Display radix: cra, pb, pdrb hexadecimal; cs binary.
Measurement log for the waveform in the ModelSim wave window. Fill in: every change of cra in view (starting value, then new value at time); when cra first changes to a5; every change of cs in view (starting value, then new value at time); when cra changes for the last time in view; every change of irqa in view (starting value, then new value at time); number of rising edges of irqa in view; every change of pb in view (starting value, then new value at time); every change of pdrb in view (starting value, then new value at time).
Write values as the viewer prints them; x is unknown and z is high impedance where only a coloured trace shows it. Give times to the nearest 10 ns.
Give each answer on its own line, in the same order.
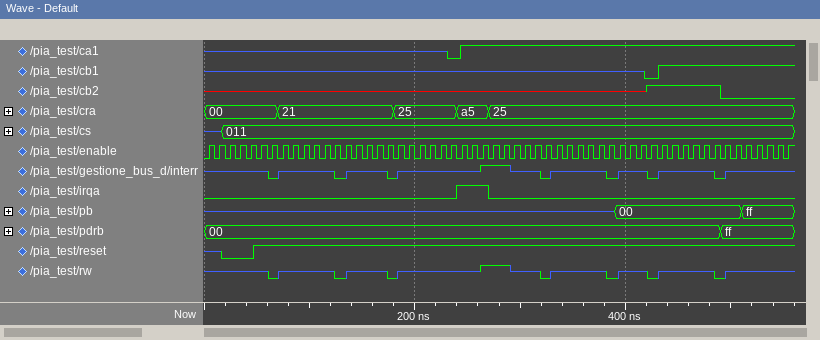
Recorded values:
00, 21 at 70 ns, 25 at 180 ns, a5 at 240 ns, 25 at 270 ns
240 ns
z, 011 at 20 ns
270 ns
0, 1 at 240 ns, 0 at 270 ns
1
z, 00 at 390 ns, ff at 510 ns
00, ff at 490 ns
